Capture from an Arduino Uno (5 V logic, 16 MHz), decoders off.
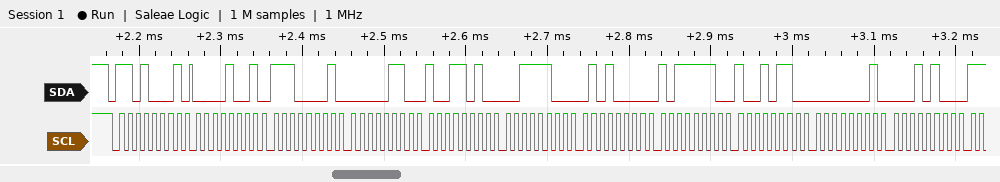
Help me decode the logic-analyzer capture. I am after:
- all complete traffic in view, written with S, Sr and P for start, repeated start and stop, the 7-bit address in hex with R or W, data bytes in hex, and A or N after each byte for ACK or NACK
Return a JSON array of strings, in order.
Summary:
["S 68R A 09 A E1 A 06 A 9A A 3C A 50 A BE A 96 A 01 A 14 A"]
